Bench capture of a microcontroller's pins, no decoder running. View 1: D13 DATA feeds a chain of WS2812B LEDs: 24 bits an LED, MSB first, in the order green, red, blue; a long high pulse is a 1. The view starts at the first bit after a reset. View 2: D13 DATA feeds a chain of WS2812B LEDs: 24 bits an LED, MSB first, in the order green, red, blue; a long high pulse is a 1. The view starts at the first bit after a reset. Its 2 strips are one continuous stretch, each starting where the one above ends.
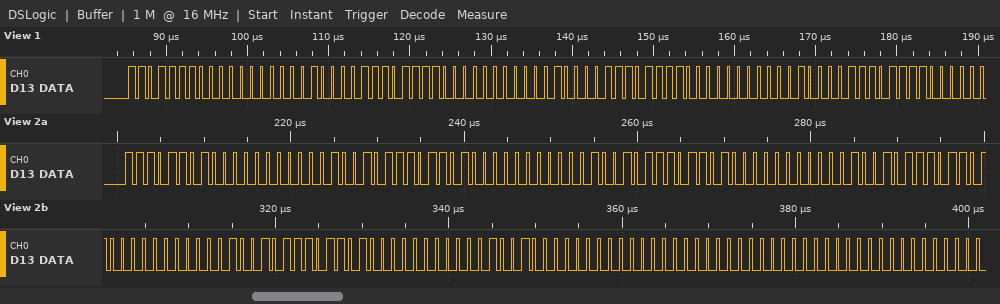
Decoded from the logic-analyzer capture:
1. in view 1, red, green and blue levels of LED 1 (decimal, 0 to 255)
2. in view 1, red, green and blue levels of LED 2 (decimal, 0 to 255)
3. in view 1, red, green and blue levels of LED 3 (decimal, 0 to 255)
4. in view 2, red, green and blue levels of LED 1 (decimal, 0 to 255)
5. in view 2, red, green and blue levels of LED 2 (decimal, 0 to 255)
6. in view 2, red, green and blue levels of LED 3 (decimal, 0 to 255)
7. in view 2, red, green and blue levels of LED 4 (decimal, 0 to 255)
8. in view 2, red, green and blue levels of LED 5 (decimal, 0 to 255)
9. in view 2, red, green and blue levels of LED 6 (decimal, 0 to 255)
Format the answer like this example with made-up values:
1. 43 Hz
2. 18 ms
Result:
1. 0, 222, 33
2. 0, 222, 33
3. 0, 222, 33
4. 0, 237, 18
5. 0, 237, 18
6. 0, 237, 18
7. 0, 237, 18
8. 0, 237, 18
9. 0, 0, 0
